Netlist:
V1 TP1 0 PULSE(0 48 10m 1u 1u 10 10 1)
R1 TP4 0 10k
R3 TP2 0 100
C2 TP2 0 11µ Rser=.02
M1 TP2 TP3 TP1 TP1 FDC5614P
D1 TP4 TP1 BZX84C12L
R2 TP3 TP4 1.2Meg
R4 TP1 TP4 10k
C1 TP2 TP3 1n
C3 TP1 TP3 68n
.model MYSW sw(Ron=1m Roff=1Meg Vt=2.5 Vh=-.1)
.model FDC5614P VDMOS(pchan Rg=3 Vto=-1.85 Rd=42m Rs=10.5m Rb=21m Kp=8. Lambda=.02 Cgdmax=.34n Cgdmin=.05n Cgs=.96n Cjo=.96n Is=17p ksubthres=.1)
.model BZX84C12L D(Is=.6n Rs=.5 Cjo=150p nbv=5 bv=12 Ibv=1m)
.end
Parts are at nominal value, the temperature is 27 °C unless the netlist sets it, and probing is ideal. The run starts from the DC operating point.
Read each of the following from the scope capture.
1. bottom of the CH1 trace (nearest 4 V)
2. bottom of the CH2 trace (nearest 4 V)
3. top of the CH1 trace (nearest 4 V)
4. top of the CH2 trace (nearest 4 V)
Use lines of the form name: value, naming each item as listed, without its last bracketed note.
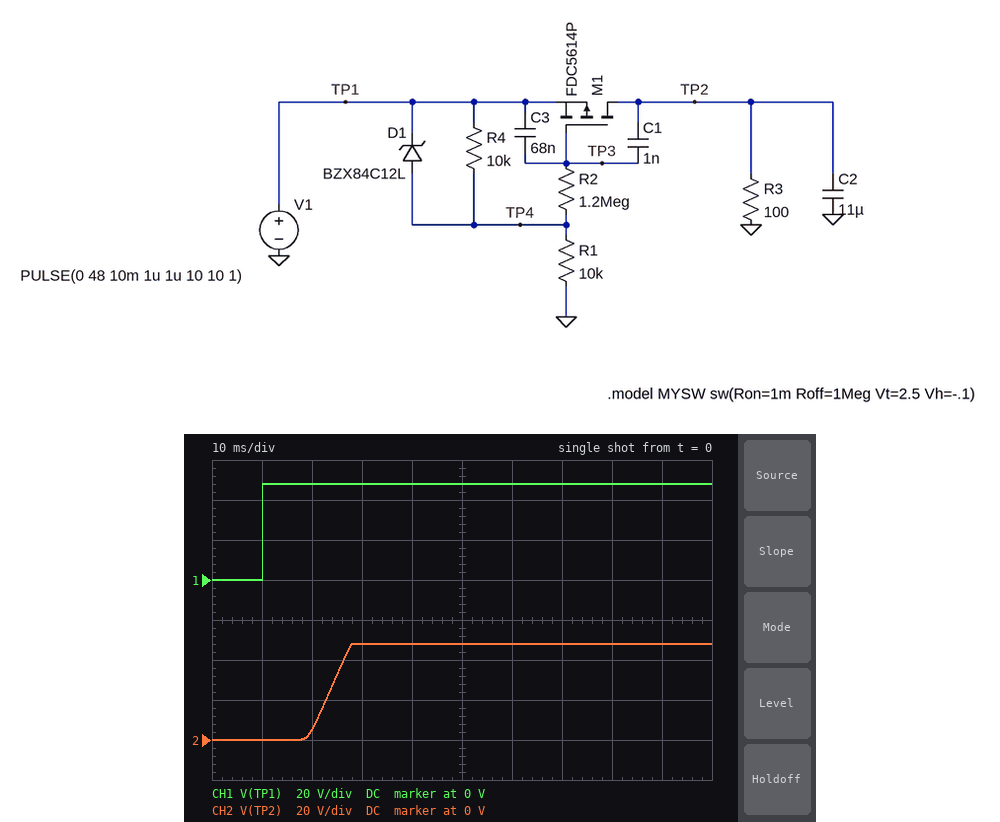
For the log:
bottom of the CH1 trace: 0 V
bottom of the CH2 trace: 0 V
top of the CH1 trace: 48 V
top of the CH2 trace: 48 V
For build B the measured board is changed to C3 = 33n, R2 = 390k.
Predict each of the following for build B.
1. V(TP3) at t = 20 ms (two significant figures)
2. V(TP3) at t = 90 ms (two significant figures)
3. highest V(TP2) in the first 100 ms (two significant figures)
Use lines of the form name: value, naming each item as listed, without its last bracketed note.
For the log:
V(TP3) at t = 20 ms: 42 V
V(TP3) at t = 90 ms: 36 V
highest V(TP2) in the first 100 ms: 48 V
